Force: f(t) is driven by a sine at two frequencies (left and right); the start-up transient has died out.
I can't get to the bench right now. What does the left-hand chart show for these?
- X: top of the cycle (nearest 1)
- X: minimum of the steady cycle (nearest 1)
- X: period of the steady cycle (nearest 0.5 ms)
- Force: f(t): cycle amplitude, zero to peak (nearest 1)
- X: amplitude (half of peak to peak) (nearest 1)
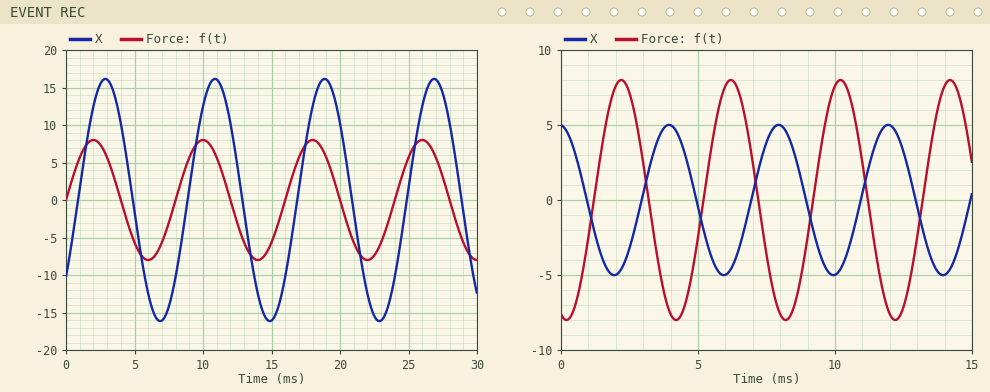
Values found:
16
-16
8.0 ms
8
16
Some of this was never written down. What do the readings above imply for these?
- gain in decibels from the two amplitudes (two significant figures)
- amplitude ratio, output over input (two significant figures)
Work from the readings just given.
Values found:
6.0 dB
2.0
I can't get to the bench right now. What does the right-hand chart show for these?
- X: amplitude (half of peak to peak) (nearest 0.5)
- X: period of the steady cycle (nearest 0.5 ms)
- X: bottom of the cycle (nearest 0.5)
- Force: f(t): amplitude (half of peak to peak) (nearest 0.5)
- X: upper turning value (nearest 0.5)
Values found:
5.0
4.0 ms
-5.0
8.0
5.0
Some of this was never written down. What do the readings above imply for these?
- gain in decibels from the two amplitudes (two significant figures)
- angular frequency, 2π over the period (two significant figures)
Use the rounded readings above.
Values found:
-4.1 dB
1.6 rad/ms
